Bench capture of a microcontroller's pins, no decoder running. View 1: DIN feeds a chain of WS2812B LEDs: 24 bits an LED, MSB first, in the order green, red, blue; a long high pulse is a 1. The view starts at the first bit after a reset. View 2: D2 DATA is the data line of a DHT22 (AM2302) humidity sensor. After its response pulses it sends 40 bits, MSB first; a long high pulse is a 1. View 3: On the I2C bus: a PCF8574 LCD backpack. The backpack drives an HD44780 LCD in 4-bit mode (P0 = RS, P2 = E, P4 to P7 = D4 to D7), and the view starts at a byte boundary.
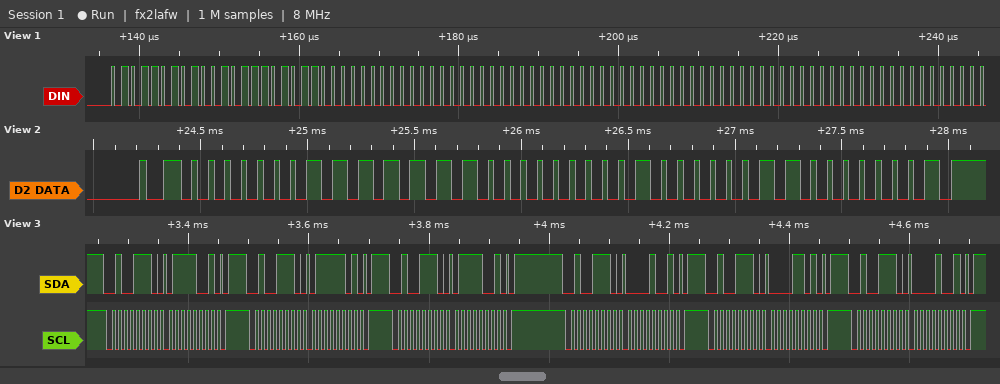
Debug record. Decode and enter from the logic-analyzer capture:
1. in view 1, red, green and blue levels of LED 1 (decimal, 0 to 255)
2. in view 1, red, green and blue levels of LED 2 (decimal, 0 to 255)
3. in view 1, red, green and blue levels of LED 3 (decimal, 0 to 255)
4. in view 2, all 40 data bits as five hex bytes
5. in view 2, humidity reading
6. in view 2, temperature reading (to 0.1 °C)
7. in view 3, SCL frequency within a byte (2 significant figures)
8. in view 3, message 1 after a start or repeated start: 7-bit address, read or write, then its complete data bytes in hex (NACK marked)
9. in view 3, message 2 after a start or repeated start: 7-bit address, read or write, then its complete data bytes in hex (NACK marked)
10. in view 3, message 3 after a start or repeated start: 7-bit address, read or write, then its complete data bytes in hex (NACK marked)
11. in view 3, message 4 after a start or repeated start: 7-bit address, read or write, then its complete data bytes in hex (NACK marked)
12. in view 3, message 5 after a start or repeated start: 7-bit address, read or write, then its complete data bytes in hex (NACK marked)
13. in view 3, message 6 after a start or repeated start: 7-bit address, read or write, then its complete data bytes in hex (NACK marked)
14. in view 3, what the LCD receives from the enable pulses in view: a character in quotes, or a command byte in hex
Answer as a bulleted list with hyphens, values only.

- 151, 90, 88
- 0, 0, 0
- 0, 0, 0
- 01 FC 01 03 01
- 50.8 %
- 25.9 °C
- 100 kHz
- 0x27 write: 79
- 0x27 write: 7D
- 0x27 write: 79
- 0x27 write: 09
- 0x27 write: 0D
- 0x27 write: 09
- 'p'
